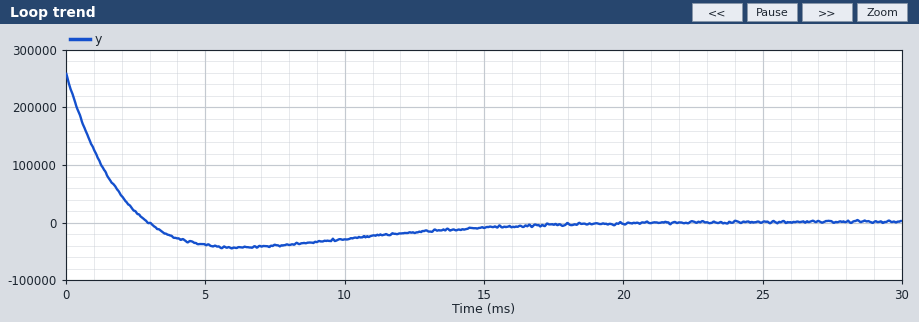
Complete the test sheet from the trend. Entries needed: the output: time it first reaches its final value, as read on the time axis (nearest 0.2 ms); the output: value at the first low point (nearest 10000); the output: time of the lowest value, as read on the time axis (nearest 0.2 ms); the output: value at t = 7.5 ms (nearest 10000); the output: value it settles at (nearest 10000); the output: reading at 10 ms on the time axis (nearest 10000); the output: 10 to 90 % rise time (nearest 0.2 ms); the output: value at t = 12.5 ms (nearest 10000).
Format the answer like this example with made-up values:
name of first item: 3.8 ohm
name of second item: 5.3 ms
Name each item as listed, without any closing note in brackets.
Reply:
the output: time it first reaches its final value, as read on the time axis: 3.0 ms
the output: value at the first low point: -40000
the output: time of the lowest value, as read on the time axis: 6.2 ms
the output: value at t = 7.5 ms: -40000
the output: value it settles at: 0
the output: reading at 10 ms on the time axis: -30000
the output: 10 to 90 % rise time: 2.2 ms
the output: value at t = 12.5 ms: -20000
